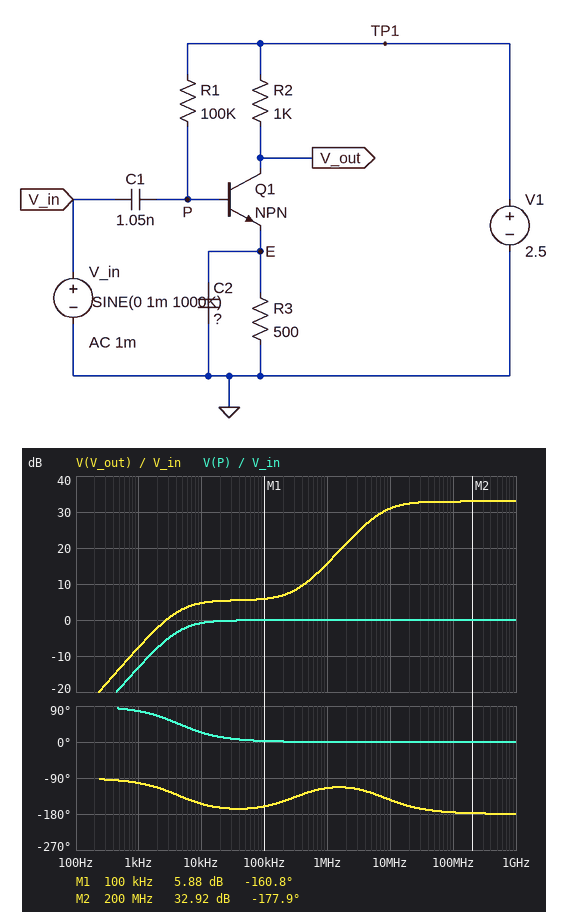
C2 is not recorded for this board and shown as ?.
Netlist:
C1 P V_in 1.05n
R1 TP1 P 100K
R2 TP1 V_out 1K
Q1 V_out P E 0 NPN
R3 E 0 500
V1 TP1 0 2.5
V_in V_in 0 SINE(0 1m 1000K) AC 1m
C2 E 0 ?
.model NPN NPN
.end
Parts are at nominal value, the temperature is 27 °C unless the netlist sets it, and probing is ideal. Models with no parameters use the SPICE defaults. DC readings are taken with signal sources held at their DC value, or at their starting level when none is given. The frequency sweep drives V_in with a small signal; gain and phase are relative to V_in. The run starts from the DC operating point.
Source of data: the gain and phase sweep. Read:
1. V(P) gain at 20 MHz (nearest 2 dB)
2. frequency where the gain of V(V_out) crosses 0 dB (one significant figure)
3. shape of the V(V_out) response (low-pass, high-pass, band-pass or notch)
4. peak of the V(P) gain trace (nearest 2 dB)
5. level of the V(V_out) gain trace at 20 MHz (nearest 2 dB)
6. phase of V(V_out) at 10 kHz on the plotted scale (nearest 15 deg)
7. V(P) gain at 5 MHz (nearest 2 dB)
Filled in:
0 dB
3 kHz
high-pass
0 dB
32 dB
-150 deg
0 dB
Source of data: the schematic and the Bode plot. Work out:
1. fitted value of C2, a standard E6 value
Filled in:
1 nF
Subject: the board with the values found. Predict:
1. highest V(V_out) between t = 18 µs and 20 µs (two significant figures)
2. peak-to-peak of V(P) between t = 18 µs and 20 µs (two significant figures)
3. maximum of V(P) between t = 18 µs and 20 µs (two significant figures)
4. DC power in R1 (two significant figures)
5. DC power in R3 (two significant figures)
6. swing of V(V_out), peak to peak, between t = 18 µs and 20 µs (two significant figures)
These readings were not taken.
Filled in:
1.4 V
2.0 mV
1.4 V
13 µW
670 µW
12 mV
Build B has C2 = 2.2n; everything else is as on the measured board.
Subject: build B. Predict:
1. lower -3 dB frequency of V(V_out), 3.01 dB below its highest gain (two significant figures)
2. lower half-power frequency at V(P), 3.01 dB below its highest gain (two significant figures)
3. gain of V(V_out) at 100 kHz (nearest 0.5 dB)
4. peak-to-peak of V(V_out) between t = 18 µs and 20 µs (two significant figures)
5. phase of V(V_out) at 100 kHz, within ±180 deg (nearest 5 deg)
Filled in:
3.4 MHz
4.5 kHz
7.0 dB
25 mV
-145 deg
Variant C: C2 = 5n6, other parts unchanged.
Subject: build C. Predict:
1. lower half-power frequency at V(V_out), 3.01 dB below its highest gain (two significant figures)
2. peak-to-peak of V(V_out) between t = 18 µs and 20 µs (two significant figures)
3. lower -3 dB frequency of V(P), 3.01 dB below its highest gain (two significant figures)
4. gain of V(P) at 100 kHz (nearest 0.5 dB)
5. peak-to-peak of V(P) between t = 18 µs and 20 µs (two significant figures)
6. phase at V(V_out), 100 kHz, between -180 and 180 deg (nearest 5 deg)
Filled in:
1.4 MHz
52 mV
4.6 kHz
-0.5 dB
1.9 mV
-120 deg
